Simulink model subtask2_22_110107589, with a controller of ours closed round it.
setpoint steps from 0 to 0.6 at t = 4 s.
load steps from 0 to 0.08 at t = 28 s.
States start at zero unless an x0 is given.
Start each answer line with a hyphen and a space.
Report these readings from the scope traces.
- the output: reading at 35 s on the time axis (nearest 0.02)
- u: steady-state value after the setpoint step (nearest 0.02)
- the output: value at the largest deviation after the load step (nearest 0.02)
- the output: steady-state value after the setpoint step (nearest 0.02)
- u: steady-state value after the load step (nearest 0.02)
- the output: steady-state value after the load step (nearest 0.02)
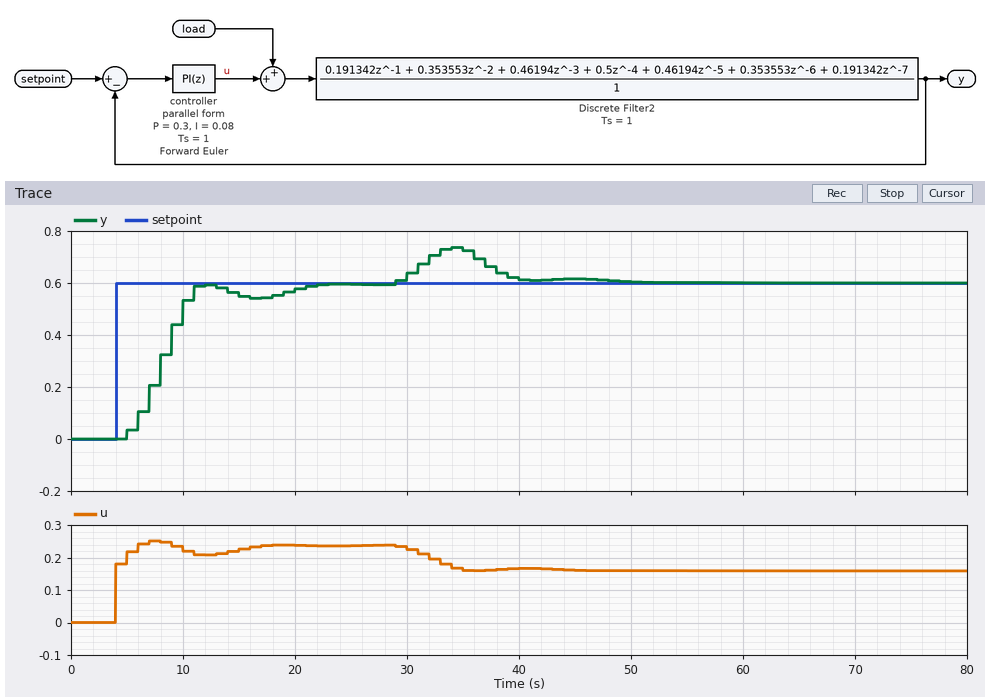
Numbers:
- 0.72
- 0.24
- 0.74
- 0.60
- 0.16
- 0.60
